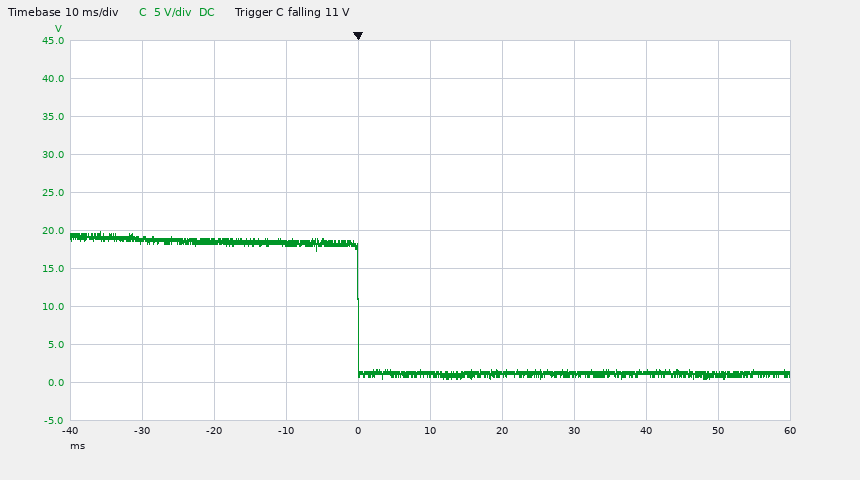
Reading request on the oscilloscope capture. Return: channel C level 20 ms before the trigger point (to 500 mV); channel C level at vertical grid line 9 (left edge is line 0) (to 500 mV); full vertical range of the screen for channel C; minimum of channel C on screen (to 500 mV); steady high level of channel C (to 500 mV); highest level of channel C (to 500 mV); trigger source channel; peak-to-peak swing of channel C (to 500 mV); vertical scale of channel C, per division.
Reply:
18.5 V
1.0 V
50 V
500 mV
18.5 V
20.0 V
channel C
19.5 V
5 V
